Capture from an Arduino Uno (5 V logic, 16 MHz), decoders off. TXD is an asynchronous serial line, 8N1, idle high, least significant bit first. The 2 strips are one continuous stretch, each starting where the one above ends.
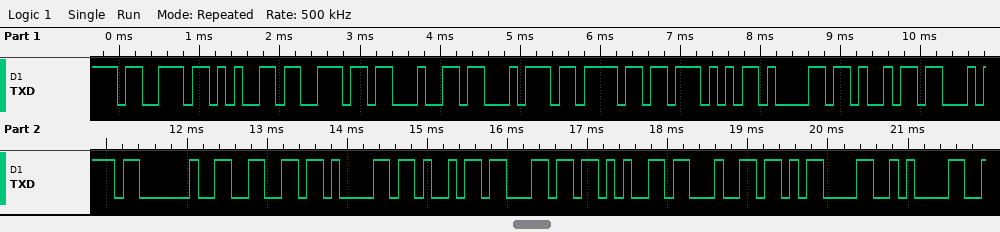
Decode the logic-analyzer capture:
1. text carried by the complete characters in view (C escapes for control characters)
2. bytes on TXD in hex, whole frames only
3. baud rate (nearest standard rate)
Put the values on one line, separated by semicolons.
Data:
"sendtoWait failed\r\n"; 0x73 0x65 0x6E 0x64 0x74 0x6F 0x57 0x61 0x69 0x74 0x20 0x66 0x61 0x69 0x6C 0x65 0x64 0x0D 0x0A; 9600 baud
